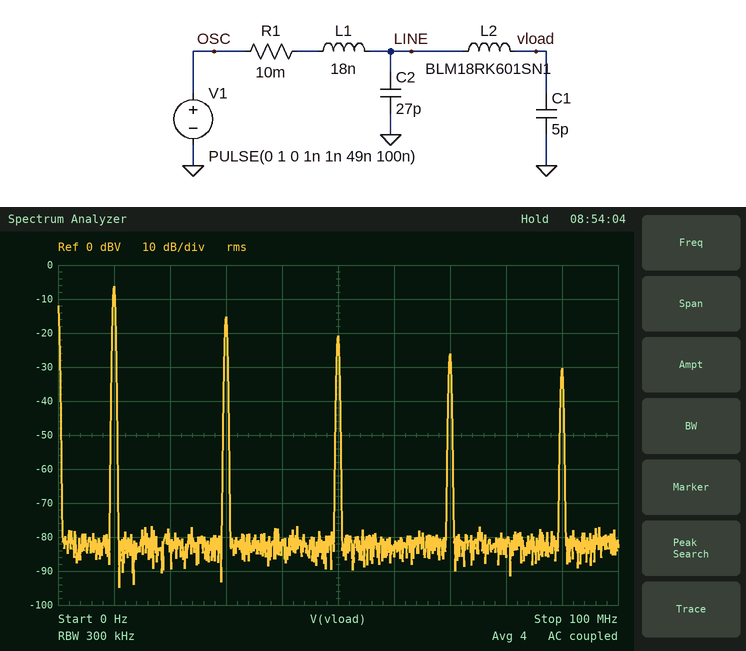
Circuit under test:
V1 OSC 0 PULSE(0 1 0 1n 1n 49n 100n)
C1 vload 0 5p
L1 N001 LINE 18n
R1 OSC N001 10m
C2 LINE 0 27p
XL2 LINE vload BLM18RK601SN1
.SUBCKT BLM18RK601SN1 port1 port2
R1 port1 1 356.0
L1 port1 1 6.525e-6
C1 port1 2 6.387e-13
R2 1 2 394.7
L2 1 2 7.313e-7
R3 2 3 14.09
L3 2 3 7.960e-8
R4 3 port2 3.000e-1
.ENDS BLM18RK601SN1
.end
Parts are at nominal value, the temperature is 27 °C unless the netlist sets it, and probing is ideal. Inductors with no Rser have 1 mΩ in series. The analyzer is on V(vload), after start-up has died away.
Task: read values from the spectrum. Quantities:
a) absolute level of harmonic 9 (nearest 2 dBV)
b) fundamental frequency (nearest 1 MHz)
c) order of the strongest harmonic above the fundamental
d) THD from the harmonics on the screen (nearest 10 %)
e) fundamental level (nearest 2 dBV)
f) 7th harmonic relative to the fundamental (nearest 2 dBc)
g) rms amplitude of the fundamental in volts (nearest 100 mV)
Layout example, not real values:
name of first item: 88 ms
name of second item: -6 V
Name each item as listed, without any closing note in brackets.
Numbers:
absolute level of harmonic 9: -30 dBV
fundamental frequency: 10 MHz
order of the strongest harmonic above the fundamental: 3
THD from the harmonics on the screen: 40 %
fundamental level: -6 dBV
7th harmonic relative to the fundamental: -20 dBc
rms amplitude of the fundamental in volts: 500 mV
